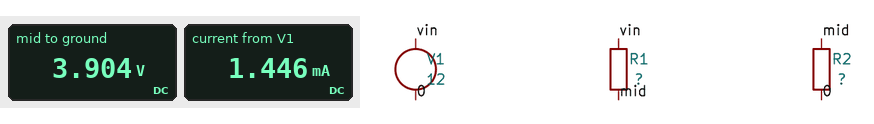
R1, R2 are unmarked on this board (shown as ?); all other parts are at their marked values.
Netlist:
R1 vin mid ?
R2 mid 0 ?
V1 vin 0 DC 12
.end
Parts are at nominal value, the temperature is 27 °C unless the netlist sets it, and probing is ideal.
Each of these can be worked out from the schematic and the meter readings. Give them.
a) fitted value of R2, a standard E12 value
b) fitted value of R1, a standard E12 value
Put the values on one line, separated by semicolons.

2.7 kΩ; 5.6 kΩ
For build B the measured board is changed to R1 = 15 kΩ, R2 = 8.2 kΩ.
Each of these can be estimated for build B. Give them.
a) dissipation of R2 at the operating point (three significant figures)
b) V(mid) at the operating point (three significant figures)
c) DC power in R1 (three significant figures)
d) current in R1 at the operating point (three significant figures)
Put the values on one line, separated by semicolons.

2.19 mW; 4.24 V; 4.01 mW; 517 µA
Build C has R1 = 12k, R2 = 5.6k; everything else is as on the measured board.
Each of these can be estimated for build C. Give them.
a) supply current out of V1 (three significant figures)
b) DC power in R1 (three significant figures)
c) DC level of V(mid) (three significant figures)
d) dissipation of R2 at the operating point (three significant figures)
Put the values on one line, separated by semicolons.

682 µA; 5.58 mW; 3.82 V; 2.60 mW
